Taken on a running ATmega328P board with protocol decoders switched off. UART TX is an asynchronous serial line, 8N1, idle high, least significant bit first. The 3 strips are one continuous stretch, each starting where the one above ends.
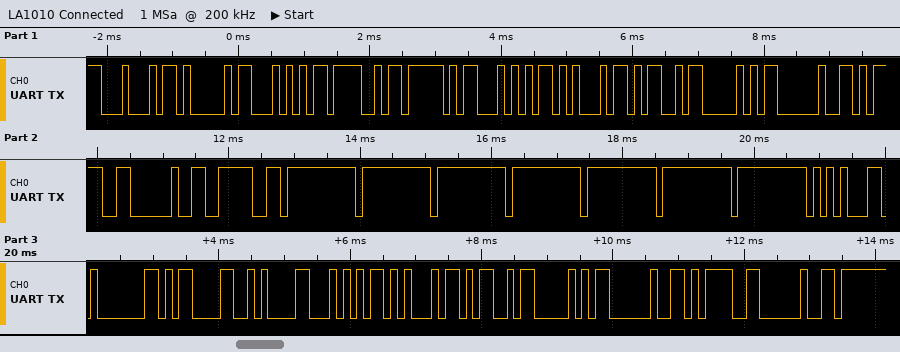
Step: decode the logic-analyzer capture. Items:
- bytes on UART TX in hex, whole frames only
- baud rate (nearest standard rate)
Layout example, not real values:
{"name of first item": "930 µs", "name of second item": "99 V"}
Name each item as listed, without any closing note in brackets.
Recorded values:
{"bytes on UART TX in hex, whole frames only": "0x44 0x41 0x54 0x4F 0x5F 0x54 0x45 0x4D 0x50 0x20 0x3D 0x20 0x3E 0xFF 0xFF 0xFF 0xFF 0xFF 0xFF 0xFF 0x15 0x01 0x0D 0x0A 0x54 0x45 0x4D 0x50 0x20 0x3D 0x20", "baud rate": "9600 baud"}
